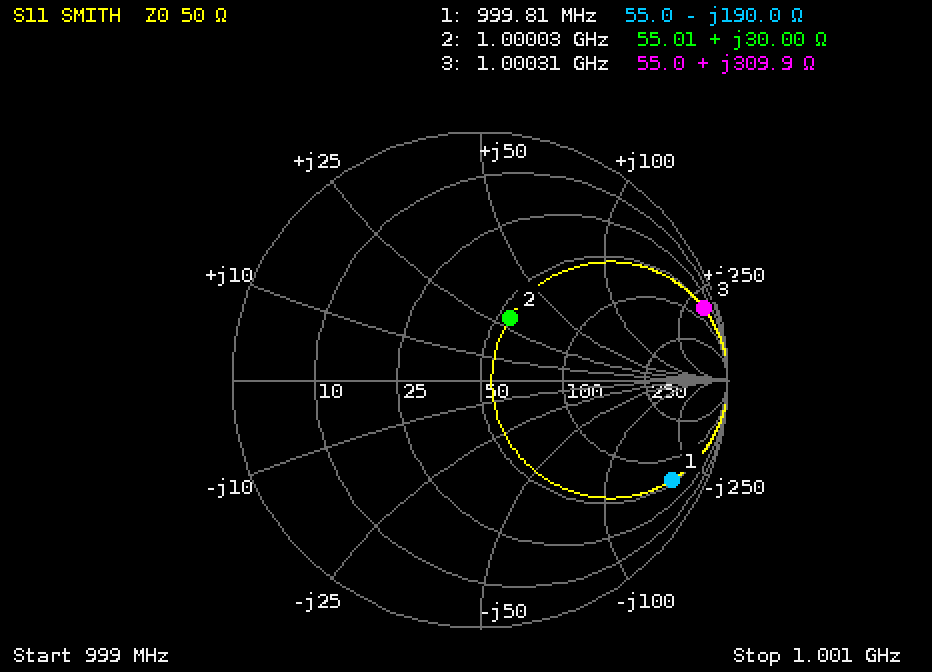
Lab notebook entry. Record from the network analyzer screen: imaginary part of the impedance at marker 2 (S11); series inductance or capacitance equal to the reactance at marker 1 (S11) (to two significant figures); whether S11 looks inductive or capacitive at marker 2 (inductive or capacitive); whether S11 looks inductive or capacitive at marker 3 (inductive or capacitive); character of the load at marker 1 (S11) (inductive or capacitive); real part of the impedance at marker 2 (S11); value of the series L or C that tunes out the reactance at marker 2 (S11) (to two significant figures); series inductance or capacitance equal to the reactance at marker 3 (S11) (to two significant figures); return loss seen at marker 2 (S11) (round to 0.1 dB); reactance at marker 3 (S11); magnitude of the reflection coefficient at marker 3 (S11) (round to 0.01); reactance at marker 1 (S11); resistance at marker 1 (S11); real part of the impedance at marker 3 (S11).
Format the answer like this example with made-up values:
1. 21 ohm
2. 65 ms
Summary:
1. +30.00 Ω
2. 840 fF
3. inductive
4. inductive
5. capacitive
6. 55.01 Ω
7. 5.3 pF
8. 49 nH
9. 11.1 dB
10. +309.9 Ω
11. 0.95
12. -190.0 Ω
13. 55.0 Ω
14. 55.0 Ω
